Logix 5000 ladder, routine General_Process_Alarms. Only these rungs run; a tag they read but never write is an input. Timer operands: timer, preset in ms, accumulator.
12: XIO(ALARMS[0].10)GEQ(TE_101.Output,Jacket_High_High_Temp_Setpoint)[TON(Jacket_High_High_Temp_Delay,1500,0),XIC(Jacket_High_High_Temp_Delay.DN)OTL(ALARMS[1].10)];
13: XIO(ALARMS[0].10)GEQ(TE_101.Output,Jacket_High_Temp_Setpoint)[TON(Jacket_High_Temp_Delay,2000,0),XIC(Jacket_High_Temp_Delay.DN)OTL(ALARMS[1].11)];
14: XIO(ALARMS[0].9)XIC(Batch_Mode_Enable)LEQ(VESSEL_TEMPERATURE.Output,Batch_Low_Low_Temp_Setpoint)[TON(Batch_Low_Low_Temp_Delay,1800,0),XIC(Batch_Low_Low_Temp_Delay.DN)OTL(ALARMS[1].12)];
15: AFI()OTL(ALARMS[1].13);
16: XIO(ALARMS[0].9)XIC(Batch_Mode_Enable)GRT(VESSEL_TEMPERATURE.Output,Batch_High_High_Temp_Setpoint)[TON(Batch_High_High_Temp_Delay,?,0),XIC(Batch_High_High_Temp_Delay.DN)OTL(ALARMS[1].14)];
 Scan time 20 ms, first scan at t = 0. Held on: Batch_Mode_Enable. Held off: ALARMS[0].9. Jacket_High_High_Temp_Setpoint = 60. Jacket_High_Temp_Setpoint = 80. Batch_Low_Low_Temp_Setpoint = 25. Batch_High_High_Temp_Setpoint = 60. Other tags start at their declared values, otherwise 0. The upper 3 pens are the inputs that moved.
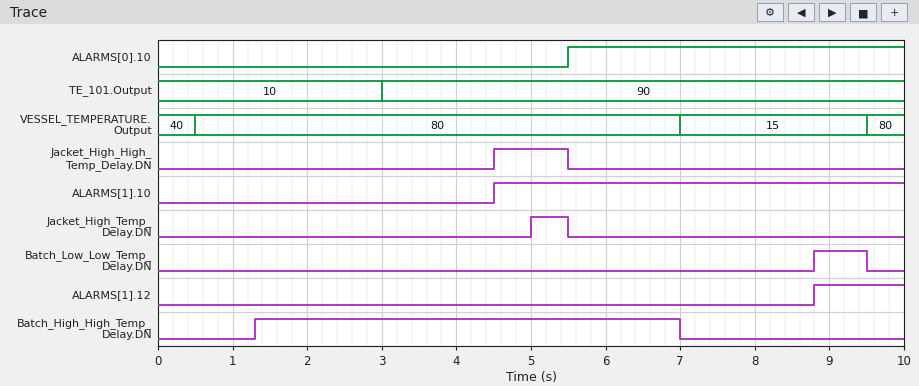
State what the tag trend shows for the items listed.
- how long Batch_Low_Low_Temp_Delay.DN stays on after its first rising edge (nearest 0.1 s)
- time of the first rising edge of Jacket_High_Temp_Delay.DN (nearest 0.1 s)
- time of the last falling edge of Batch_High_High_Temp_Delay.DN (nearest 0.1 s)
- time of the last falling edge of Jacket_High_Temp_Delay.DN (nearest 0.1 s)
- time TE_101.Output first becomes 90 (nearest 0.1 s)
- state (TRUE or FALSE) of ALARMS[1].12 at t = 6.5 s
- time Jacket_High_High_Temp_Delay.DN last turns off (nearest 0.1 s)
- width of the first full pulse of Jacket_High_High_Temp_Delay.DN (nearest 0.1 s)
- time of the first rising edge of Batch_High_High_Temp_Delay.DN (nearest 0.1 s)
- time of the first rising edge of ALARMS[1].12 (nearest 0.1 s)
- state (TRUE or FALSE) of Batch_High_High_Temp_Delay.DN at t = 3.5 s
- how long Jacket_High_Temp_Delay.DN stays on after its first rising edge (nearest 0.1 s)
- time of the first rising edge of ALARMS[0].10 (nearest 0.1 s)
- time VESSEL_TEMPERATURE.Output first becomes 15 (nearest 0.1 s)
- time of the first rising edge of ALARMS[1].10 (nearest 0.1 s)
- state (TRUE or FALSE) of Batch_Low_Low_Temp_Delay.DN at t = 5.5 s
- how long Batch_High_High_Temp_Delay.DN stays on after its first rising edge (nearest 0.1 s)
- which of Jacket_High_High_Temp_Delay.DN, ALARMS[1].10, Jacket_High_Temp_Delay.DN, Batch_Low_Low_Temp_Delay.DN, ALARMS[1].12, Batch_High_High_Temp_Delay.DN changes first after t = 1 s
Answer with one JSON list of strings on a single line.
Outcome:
["0.7 s", "5.0 s", "7.0 s", "5.5 s", "3.0 s", "FALSE", "5.5 s", "1.0 s", "1.3 s", "8.8 s", "TRUE", "0.5 s", "5.5 s", "7.0 s", "4.5 s", "FALSE", "5.7 s", "Batch_High_High_Temp_Delay.DN"]
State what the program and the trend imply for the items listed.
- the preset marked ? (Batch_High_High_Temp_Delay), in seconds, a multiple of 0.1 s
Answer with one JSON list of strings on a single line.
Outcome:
["0.8 s"]
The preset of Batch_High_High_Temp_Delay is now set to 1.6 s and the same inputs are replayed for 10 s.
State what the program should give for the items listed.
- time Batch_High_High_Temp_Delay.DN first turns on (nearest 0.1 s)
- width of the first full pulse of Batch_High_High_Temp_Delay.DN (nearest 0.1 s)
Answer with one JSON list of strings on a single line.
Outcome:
["2.1 s", "4.9 s"]
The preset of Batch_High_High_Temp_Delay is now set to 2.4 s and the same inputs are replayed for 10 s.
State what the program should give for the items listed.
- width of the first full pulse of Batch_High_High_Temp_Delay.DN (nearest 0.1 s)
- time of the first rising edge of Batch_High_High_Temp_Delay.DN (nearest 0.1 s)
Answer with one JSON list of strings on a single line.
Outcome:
["4.1 s", "2.9 s"]
